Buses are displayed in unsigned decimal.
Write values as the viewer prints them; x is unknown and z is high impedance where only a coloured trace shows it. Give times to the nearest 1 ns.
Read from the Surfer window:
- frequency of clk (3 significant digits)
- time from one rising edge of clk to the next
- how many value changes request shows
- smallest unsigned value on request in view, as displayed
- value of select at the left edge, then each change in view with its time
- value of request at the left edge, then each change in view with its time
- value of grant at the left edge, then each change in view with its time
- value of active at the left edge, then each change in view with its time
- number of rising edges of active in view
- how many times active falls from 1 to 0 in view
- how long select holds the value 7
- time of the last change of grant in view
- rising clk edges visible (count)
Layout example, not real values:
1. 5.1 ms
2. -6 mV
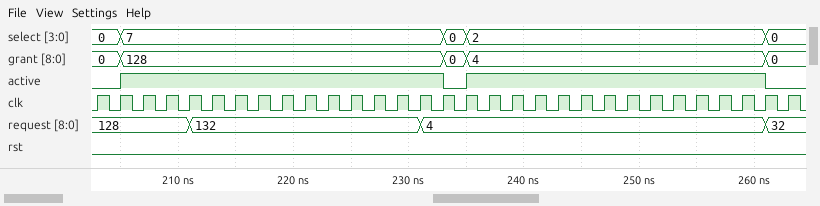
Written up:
1. 500 MHz
2. 2 ns
3. 3
4. 4
5. 0, 7 at 205 ns, 0 at 233 ns, 2 at 235 ns, 0 at 261 ns
6. 128, 132 at 211 ns, 4 at 231 ns, 32 at 261 ns
7. 0, 128 at 205 ns, 0 at 233 ns, 4 at 235 ns, 0 at 261 ns
8. 0, 1 at 205 ns, 0 at 233 ns, 1 at 235 ns, 0 at 261 ns
9. 2
10. 2
11. 28 ns
12. 261 ns
13. 31
